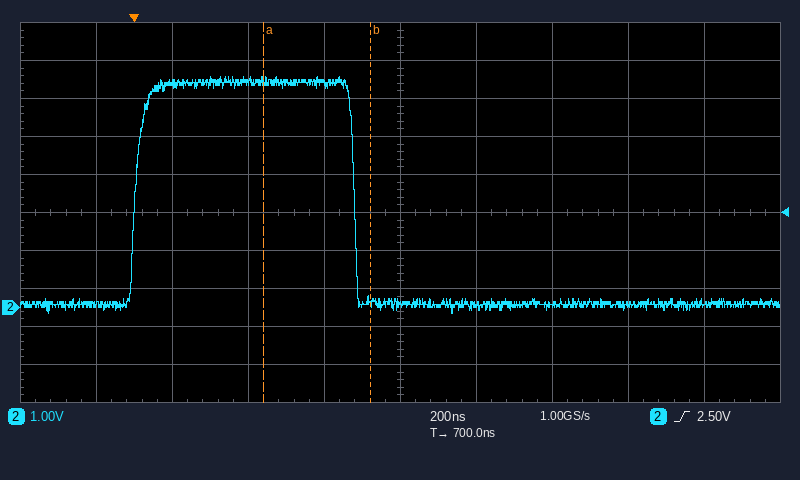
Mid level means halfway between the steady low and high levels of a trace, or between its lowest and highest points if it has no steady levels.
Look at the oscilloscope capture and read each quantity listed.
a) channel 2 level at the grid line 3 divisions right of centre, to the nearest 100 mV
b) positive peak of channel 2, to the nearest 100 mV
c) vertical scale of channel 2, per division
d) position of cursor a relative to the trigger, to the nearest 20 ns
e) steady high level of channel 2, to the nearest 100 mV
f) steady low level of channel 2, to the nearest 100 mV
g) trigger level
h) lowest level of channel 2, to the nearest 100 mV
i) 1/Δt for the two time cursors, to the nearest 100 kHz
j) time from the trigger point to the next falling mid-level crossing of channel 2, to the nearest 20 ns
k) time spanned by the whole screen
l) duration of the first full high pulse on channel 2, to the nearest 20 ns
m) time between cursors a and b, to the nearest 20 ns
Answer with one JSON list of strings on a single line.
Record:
["100 mV", "6.1 V", "1 V", "+340 ns", "5.9 V", "100 mV", "2.50 V", "-200 mV", "3.6 MHz", "580 ns", "2 µs", "580 ns", "280 ns"]
